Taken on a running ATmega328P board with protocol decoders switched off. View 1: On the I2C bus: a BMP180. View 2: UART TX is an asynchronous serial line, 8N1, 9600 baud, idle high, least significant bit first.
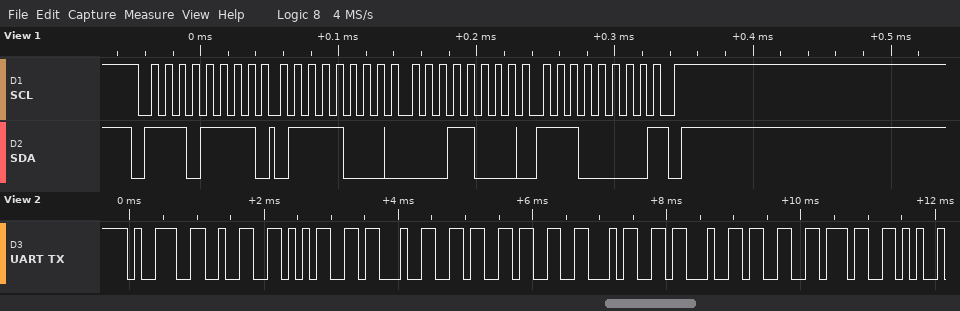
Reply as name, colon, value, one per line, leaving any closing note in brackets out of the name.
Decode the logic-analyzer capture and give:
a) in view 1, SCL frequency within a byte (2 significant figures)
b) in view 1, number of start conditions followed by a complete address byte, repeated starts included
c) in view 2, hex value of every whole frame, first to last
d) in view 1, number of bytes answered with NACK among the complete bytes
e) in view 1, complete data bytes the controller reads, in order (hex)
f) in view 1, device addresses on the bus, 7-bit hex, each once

in view 1, SCL frequency within a byte: 100 kHz
in view 1, number of start conditions followed by a complete address byte, repeated starts included: 1
in view 2, hex value of every whole frame, first to last: 39 32 35 23 36 33 34 23 33 37
in view 1, number of bytes answered with NACK among the complete bytes: 1
in view 1, complete data bytes the controller reads, in order: 78 18 E0
in view 1, device addresses on the bus, 7-bit hex, each once: 0x77
